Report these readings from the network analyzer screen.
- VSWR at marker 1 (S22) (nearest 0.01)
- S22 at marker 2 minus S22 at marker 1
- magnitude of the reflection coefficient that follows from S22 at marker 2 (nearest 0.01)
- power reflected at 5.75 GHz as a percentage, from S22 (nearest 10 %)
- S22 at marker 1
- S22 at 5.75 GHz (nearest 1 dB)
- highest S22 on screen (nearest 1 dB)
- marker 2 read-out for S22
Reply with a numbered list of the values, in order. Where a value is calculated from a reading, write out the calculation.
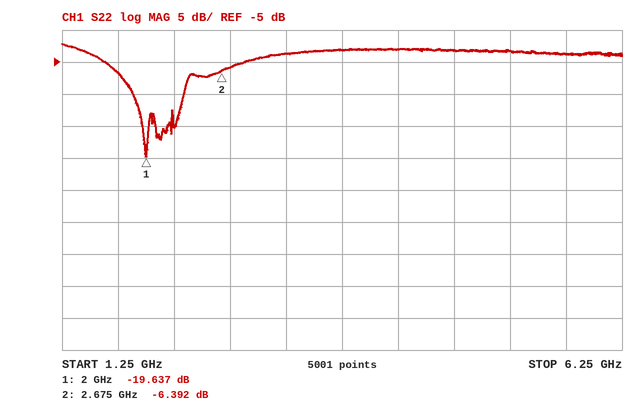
1. (1 + 0.1043)/(1 − 0.1043) ≈ 1.23
2. -6.392 − (-19.637) = 13.245 dB
3. 10^(-6.392/20) ≈ 0.48
4. 10^(-4/10) ≈ 40 %
5. -19.637 dB
6. -4 dB
7. -2 dB
8. -6.392 dB
